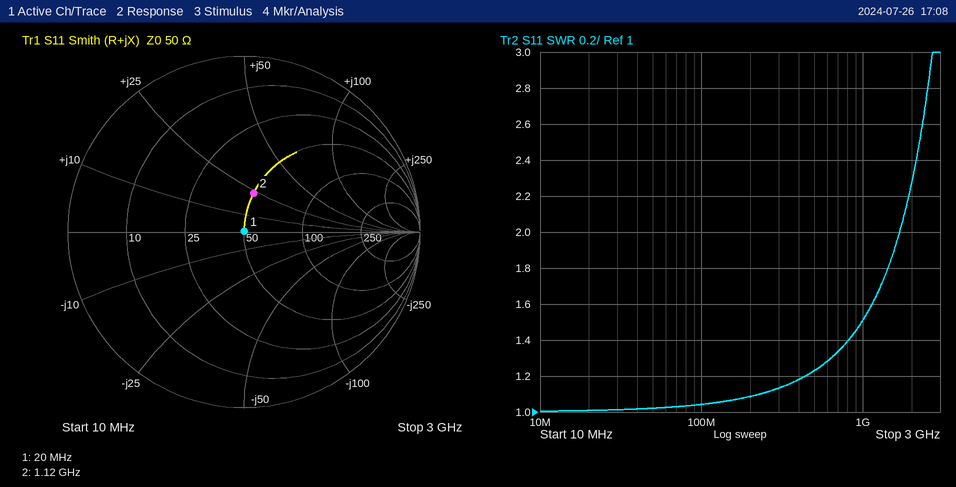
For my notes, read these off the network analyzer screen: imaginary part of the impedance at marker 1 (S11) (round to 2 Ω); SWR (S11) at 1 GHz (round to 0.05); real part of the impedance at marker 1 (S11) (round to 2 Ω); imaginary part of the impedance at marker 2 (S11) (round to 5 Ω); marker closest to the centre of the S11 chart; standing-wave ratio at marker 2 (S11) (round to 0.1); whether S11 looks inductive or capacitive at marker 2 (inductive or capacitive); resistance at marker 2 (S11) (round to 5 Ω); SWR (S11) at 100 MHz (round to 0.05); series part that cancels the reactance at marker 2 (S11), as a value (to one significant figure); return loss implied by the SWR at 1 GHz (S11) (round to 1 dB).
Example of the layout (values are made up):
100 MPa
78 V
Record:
0 Ω
1.50
50 Ω
+25 Ω
marker 1
1.6
inductive
50 Ω
1.05
6 pF
14 dB
